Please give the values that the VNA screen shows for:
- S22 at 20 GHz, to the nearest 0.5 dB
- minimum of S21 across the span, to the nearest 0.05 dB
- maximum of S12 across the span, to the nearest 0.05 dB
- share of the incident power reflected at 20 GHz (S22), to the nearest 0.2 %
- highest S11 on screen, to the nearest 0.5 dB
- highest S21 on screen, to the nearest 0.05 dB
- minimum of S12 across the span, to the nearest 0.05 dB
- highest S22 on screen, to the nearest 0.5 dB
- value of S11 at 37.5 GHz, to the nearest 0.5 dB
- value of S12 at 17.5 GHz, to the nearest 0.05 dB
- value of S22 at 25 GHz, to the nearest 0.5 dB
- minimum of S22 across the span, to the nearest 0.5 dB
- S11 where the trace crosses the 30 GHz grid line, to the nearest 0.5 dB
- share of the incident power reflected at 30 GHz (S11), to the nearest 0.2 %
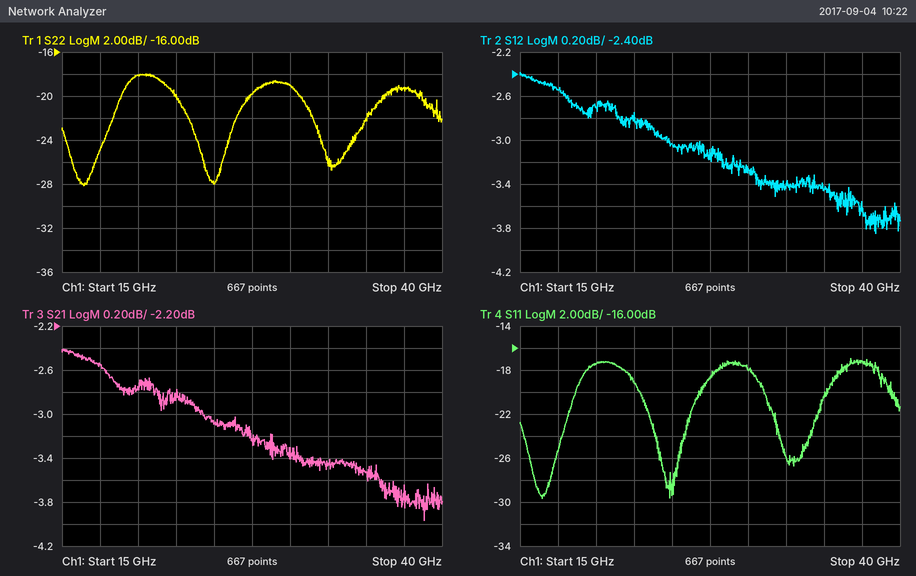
-18.0 dB
-3.95 dB
-2.40 dB
1.6 %
-17.0 dB
-2.40 dB
-3.85 dB
-18.0 dB
-17.0 dB
-2.55 dB
-28.0 dB
-28.0 dB
-18.0 dB
1.6 %
